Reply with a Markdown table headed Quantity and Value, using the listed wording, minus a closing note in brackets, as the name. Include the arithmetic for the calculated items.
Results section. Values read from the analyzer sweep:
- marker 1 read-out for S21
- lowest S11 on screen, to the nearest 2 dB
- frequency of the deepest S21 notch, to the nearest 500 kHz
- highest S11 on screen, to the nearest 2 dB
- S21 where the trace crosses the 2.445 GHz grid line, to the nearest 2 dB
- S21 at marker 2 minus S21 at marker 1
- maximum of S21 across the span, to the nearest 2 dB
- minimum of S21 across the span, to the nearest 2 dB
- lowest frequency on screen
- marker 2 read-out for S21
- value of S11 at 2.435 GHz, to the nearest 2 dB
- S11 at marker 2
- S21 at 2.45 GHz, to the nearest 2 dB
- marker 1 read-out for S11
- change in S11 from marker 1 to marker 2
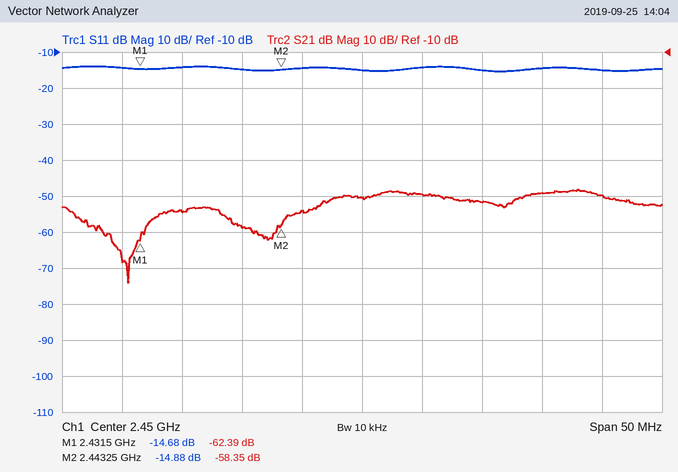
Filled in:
| Quantity | Value |
|---|---|
| marker 1 read-out for S21 | -62.39 dB |
| lowest S11 on screen, to the nearest 2 dB | -16 dB |
| frequency of the deepest S21 notch, to the nearest 500 kHz | 2.4305 GHz |
| highest S11 on screen, to the nearest 2 dB | -14 dB |
| S21 where the trace crosses the 2.445 GHz grid line, to the nearest 2 dB | -54 dB |
| S21 at marker 2 minus S21 at marker 1 | -58.35 − (-62.39) = 4.04 dB |
| maximum of S21 across the span, to the nearest 2 dB | -48 dB |
| minimum of S21 across the span, to the nearest 2 dB | -74 dB |
| lowest frequency on screen | 2.425 GHz |
| marker 2 read-out for S21 | -58.35 dB |
| value of S11 at 2.435 GHz, to the nearest 2 dB | -14 dB |
| S11 at marker 2 | -14.88 dB |
| S21 at 2.45 GHz, to the nearest 2 dB | -50 dB |
| marker 1 read-out for S11 | -14.68 dB |
| change in S11 from marker 1 to marker 2 | -14.88 − (-14.68) = -0.20 dB |
